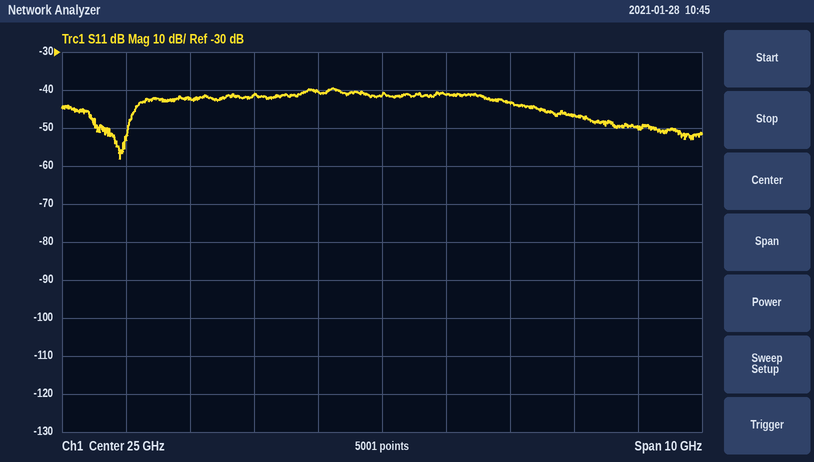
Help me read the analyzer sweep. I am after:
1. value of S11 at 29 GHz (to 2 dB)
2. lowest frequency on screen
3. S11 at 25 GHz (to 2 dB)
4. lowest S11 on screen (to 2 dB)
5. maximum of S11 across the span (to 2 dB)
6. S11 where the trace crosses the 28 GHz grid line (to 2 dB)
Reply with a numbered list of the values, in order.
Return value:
1. -50 dB
2. 20 GHz
3. -42 dB
4. -58 dB
5. -40 dB
6. -46 dB
